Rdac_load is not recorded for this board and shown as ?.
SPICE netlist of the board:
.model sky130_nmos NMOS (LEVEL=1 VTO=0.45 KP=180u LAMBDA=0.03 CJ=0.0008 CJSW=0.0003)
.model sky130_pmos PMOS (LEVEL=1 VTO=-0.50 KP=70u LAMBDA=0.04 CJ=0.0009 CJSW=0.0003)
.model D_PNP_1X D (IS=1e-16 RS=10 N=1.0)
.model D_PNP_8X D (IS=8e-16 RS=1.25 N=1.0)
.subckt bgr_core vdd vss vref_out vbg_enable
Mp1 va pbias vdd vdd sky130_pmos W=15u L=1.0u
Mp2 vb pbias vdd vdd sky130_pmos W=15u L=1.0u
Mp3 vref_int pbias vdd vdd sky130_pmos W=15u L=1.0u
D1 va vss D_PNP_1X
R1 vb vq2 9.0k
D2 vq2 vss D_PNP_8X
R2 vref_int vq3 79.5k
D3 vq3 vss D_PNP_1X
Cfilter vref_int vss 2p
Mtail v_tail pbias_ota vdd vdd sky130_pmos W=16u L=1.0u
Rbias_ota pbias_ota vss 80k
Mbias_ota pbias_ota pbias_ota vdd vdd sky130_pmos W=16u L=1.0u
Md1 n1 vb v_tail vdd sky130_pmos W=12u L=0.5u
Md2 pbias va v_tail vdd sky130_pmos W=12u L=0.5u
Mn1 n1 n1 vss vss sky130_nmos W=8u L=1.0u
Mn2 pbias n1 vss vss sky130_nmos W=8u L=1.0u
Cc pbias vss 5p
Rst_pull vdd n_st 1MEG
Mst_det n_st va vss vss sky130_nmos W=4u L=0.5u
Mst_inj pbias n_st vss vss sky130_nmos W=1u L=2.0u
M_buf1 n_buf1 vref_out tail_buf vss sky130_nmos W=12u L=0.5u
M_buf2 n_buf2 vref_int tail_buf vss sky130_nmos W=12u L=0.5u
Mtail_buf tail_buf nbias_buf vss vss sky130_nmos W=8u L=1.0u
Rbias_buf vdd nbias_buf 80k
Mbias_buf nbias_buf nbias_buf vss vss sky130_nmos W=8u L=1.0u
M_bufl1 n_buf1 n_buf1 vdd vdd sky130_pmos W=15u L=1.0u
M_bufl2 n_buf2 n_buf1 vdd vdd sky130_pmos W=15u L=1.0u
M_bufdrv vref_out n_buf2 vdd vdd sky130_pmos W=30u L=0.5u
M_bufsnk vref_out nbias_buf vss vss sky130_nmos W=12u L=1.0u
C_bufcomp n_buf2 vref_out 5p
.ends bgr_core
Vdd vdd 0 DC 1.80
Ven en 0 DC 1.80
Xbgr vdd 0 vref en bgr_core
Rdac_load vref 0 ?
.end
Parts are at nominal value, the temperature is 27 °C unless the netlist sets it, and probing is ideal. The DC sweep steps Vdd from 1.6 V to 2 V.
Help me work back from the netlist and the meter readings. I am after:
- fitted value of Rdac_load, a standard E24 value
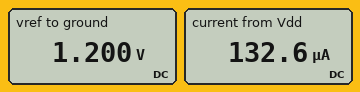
43 kΩ
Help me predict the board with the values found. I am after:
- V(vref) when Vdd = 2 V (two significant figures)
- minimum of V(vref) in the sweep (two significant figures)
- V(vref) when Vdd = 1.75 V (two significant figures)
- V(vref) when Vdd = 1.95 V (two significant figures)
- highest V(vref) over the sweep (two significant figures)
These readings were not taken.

1.8 V
1.1 V
1.1 V
1.7 V
1.8 V
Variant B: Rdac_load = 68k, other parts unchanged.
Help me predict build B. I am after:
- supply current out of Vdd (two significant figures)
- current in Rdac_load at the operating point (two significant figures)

120 µA
18 µA
